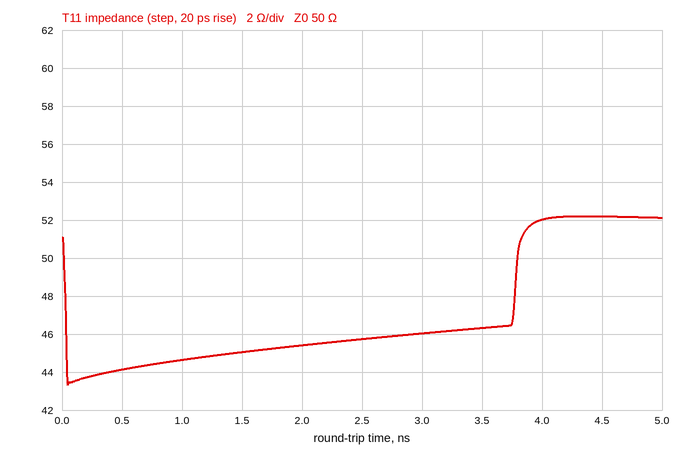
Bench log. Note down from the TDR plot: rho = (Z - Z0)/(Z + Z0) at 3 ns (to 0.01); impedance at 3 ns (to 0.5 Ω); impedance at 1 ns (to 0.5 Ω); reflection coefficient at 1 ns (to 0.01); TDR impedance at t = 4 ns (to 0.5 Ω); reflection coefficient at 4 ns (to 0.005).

-0.04
46.0 Ω
44.5 Ω
-0.06
52.0 Ω
+0.020
